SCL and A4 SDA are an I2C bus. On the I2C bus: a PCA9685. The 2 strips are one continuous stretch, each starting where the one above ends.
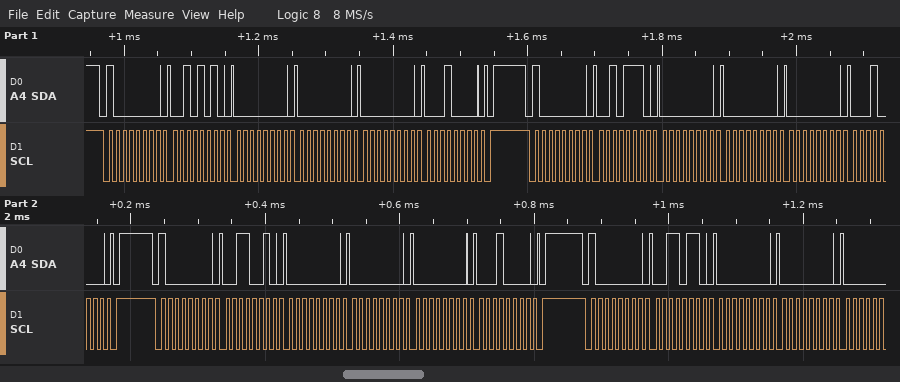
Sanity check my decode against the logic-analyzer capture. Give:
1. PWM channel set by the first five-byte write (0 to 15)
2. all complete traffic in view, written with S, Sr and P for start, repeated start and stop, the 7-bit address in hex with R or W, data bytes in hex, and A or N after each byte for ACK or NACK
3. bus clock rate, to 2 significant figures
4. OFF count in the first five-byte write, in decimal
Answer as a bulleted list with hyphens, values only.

- 9
- S 40W A 2A A 00 A 00 A 00 A 10 A P S 40W A 2E A 00 A 00 A 00 A 10 A P S 40W A 32 A 00 A 00 A 00 A 10 A P S 40W A 36 A 00 A 00 A
- 100 kHz
- 4096
